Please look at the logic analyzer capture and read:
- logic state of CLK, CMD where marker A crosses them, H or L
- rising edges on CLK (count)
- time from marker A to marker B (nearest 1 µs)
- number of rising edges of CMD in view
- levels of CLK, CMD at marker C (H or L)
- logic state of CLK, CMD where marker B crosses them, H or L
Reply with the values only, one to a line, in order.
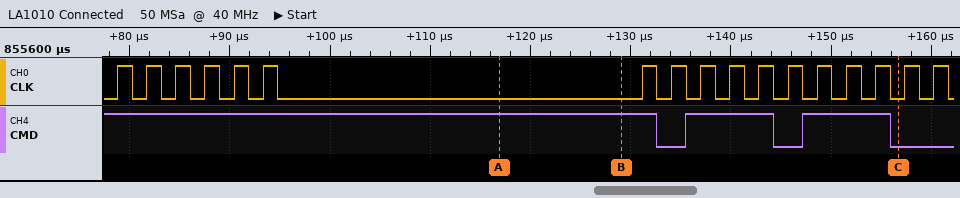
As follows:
CLK=L, CMD=H
17
12 µs
2
CLK=L, CMD=L
CLK=L, CMD=H
